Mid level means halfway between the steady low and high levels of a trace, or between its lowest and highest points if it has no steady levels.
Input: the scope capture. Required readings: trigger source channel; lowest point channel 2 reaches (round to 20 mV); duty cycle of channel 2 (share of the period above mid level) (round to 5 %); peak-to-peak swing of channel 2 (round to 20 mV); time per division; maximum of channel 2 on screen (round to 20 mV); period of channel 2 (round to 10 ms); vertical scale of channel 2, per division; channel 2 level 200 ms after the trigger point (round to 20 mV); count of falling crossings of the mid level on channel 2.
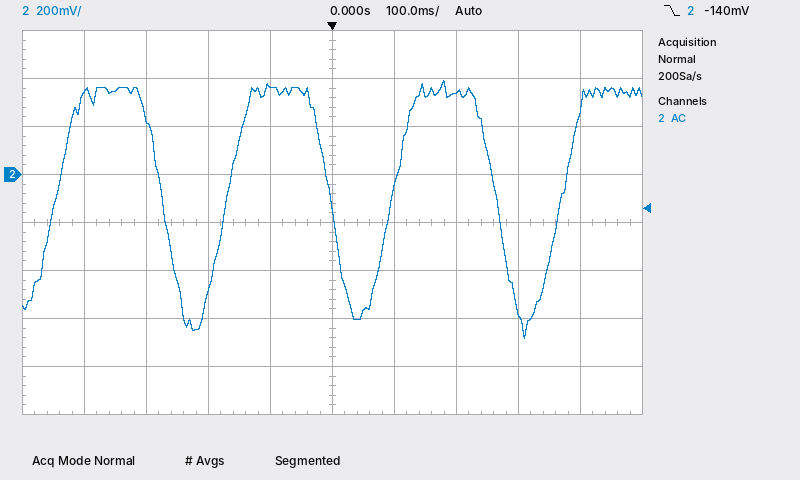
channel 2
-680 mV
65 %
1.08 V
100 ms
400 mV
270 ms
200 mV
340 mV
3
